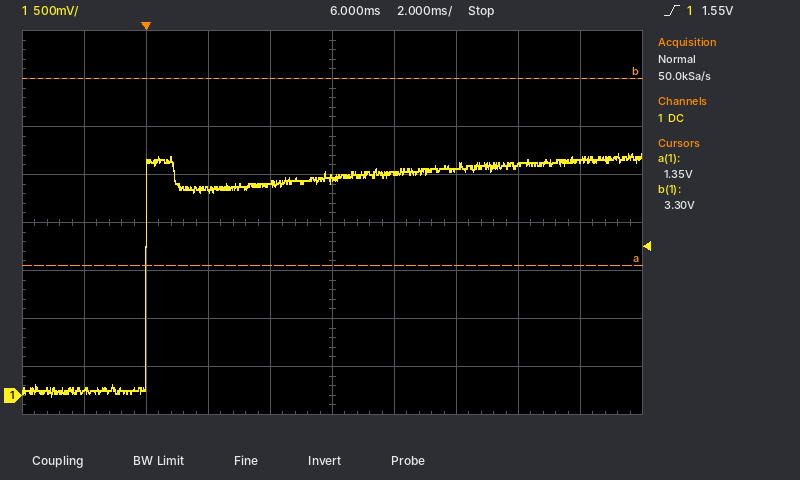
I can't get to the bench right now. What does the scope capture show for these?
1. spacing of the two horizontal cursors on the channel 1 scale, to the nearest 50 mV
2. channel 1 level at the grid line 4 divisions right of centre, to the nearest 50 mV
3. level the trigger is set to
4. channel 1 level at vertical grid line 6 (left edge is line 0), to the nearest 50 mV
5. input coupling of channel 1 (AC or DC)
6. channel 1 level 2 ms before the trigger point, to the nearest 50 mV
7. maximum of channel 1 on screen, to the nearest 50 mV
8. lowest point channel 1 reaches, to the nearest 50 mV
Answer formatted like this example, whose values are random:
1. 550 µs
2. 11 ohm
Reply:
1. 1.95 V
2. 2.45 V
3. 1.55 V
4. 2.30 V
5. DC
6. 50 mV
7. 2.50 V
8. 0 mV
